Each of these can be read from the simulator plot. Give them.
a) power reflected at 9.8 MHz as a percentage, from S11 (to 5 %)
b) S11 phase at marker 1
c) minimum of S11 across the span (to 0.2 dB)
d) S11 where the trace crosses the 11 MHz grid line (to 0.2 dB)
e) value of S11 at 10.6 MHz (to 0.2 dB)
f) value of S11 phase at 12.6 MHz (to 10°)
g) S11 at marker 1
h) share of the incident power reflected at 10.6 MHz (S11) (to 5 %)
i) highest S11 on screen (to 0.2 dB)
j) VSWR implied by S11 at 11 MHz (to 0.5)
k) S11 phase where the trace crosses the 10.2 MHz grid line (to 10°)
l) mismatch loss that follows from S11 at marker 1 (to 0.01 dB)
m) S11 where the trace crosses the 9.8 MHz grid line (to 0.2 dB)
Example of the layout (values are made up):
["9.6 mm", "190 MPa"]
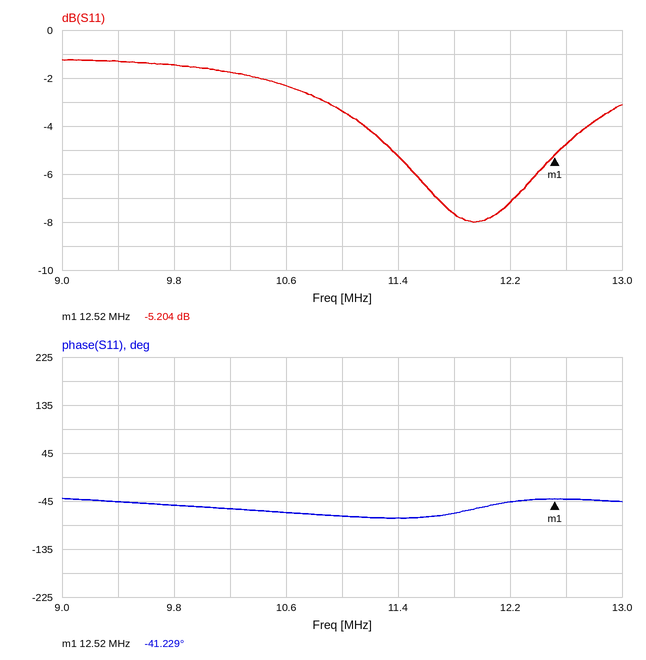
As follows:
["70 %", "-41.229°", "-8.0 dB", "-3.4 dB", "-2.4 dB", "-40°", "-5.204 dB", "60 %", "-1.2 dB", "5.0", "-60°", "1.56 dB", "-1.4 dB"]
